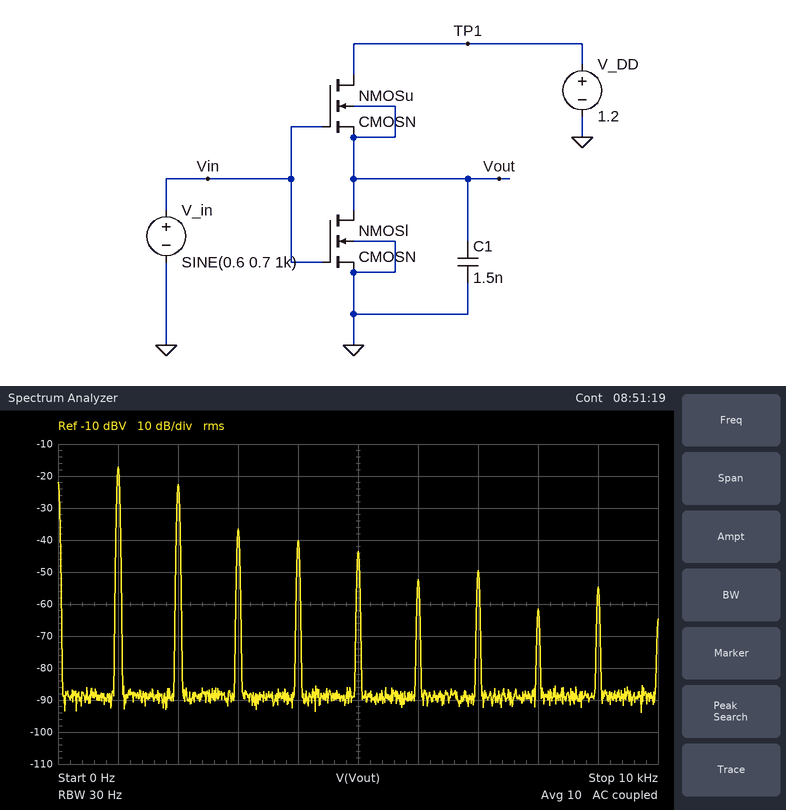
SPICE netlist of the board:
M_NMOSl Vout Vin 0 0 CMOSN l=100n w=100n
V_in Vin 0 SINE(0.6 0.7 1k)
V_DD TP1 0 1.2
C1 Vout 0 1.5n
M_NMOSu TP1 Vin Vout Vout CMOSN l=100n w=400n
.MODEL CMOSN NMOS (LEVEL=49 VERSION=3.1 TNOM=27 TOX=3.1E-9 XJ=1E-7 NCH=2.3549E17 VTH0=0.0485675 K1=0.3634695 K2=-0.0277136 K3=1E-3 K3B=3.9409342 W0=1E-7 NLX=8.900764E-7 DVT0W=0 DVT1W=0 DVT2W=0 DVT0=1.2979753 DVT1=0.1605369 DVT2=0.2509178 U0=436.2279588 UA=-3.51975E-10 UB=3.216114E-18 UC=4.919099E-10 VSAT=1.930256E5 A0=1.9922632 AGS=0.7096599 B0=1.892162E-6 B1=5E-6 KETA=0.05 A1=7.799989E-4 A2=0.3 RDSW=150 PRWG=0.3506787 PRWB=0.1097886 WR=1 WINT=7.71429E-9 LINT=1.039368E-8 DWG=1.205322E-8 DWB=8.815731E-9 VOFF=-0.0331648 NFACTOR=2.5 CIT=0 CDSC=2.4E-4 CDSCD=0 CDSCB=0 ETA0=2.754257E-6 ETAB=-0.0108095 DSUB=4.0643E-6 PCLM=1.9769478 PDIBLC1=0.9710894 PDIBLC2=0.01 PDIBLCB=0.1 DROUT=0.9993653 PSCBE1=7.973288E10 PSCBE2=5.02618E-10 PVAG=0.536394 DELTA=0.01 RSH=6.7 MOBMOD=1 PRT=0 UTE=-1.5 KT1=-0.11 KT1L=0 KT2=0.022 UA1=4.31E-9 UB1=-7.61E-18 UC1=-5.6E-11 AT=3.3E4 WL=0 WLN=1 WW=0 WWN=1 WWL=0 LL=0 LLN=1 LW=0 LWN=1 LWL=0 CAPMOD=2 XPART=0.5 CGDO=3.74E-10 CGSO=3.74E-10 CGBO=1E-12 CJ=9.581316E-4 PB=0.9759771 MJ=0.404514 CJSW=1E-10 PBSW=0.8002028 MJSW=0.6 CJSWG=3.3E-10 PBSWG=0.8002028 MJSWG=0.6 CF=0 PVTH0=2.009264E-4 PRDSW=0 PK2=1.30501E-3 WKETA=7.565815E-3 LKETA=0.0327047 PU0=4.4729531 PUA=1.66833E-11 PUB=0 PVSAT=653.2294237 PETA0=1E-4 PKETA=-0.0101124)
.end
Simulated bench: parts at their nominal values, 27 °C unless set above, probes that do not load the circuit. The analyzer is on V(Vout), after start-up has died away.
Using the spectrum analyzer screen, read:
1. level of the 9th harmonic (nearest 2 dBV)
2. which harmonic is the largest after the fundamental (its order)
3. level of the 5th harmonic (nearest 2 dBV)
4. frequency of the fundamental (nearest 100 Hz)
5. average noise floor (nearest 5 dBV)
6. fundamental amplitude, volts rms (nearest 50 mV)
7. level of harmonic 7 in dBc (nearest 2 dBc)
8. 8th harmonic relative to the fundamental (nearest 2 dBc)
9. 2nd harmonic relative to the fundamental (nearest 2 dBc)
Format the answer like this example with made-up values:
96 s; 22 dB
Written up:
-54 dBV; 2; -44 dBV; 1.0 kHz; -90 dBV; 150 mV; -32 dBc; -44 dBc; -6 dBc
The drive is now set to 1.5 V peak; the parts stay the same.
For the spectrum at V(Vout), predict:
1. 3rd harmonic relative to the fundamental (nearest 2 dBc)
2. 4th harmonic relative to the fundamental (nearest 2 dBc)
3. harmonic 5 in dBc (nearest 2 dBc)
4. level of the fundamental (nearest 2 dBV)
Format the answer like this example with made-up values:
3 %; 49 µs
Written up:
-36 dBc; -18 dBc; -24 dBc; -10 dBV
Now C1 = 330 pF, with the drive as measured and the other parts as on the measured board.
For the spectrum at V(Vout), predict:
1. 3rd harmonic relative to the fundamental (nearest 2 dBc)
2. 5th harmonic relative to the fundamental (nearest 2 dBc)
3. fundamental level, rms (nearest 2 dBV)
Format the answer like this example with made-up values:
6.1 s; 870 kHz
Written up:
-22 dBc; -30 dBc; -16 dBV
